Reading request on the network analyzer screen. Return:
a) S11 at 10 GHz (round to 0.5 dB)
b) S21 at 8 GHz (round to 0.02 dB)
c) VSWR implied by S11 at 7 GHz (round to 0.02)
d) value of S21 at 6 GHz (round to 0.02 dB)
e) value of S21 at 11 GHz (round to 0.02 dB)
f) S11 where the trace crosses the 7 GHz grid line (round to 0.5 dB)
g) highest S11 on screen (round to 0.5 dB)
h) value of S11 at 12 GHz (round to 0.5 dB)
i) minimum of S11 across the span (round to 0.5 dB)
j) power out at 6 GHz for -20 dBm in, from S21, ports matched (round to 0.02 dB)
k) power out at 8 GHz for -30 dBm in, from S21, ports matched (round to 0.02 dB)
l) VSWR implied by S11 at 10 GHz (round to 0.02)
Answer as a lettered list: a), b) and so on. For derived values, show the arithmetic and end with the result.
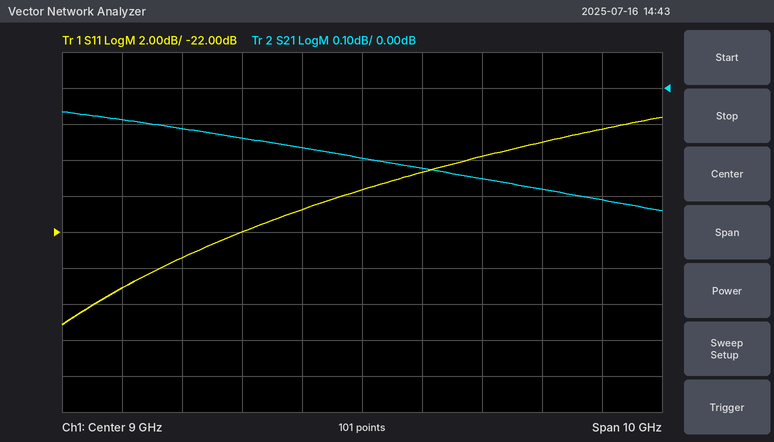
a) -18.5 dB
b) -0.16 dB
c) |Γ| = 10^(-22/20) = 0.0794; VSWR = (1 + 0.0794)/(1 − 0.0794) ≈ 1.17, so 1.18 to the nearest 0.02
d) -0.12 dB
e) -0.26 dB
f) -22.0 dB
g) -15.5 dB
h) -17.0 dB
i) -27.0 dB
j) -20 dBm + (-0.12 dB) = -20.12 dBm
k) -30 dBm + (-0.16 dB) = -30.16 dBm
l) |Γ| = 10^(-18.5/20) = 0.1189; VSWR = (1 + 0.1189)/(1 − 0.1189) ≈ 1.27, so 1.26 to the nearest 0.02
